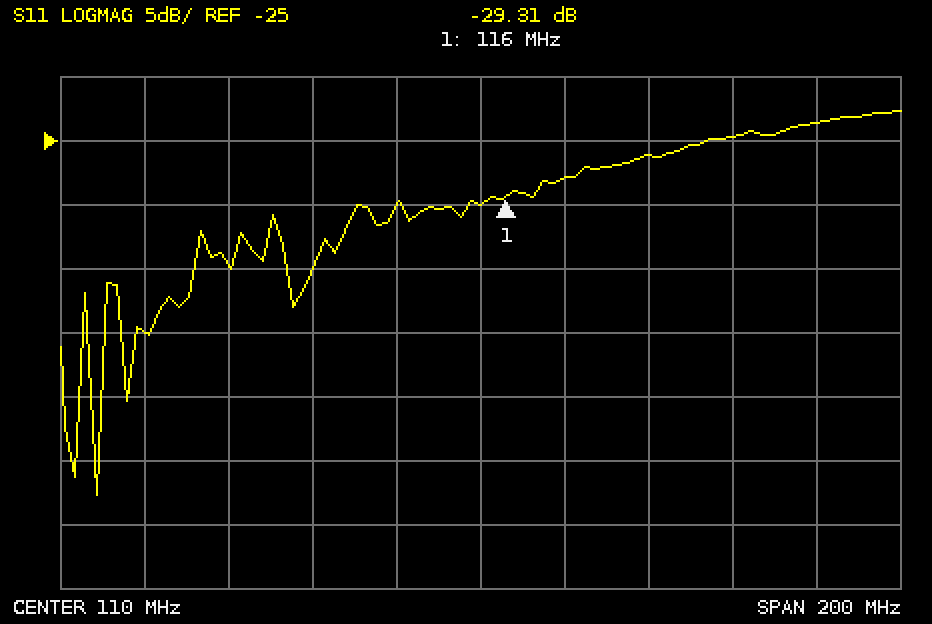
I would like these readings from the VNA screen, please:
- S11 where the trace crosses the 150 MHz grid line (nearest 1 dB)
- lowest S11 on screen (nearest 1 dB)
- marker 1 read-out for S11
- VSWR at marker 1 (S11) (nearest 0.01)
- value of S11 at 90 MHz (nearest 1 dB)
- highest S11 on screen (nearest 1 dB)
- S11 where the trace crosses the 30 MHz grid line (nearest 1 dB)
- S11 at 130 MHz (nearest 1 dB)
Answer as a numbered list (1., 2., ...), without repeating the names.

1. -26 dB
2. -53 dB
3. -29.31 dB
4. 1.07
5. -30 dB
6. -23 dB
7. -40 dB
8. -28 dB
